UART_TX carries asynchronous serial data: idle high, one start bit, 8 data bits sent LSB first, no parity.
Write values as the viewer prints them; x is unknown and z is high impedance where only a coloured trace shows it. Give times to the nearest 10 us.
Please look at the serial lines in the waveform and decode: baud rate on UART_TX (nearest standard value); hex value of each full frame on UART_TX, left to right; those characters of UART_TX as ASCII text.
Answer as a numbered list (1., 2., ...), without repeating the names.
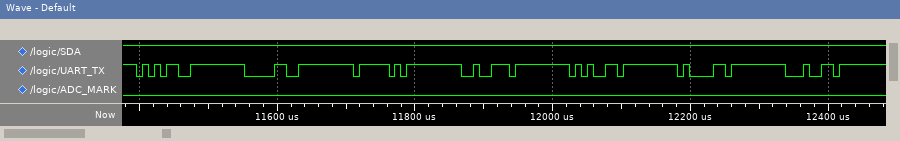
1. 115200 baud
2. 35, 30, 5F, 72, 65, 61, 64
3. "50_read"
